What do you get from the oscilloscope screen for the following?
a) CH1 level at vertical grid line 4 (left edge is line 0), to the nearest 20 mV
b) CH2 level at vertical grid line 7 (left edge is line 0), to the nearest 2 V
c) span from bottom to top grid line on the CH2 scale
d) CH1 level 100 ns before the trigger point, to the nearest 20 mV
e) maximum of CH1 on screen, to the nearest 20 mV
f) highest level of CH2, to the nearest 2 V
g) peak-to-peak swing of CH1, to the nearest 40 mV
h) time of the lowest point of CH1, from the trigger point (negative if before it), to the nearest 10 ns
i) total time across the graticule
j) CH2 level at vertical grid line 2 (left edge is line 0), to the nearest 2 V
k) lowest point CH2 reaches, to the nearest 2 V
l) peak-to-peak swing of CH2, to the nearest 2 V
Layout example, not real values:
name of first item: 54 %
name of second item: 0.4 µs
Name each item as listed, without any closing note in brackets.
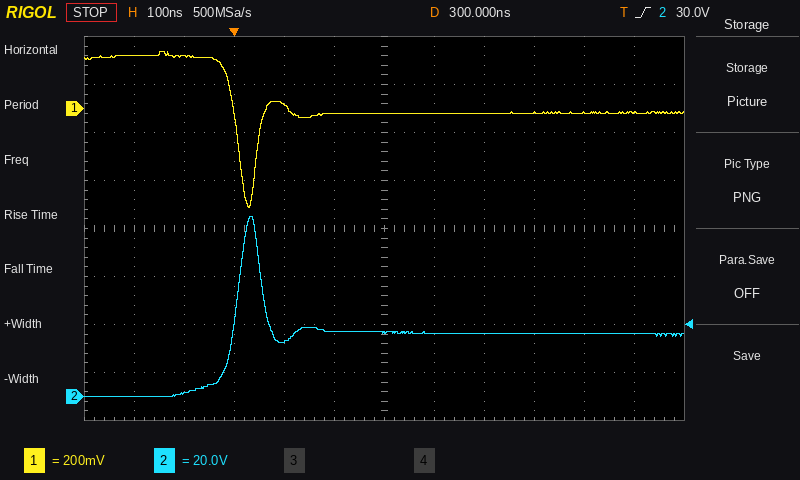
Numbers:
CH1 level at vertical grid line 4 (left edge is line 0), to the nearest 20 mV: 20 mV
CH2 level at vertical grid line 7 (left edge is line 0), to the nearest 2 V: 26 V
span from bottom to top grid line on the CH2 scale: 160 V
CH1 level 100 ns before the trigger point, to the nearest 20 mV: 220 mV
maximum of CH1 on screen, to the nearest 20 mV: 240 mV
highest level of CH2, to the nearest 2 V: 76 V
peak-to-peak swing of CH1, to the nearest 40 mV: 640 mV
time of the lowest point of CH1, from the trigger point (negative if before it), to the nearest 10 ns: +30 ns
total time across the graticule: 1.2 µs
CH2 level at vertical grid line 2 (left edge is line 0), to the nearest 2 V: 2 V
lowest point CH2 reaches, to the nearest 2 V: 0 V
peak-to-peak swing of CH2, to the nearest 2 V: 76 V
